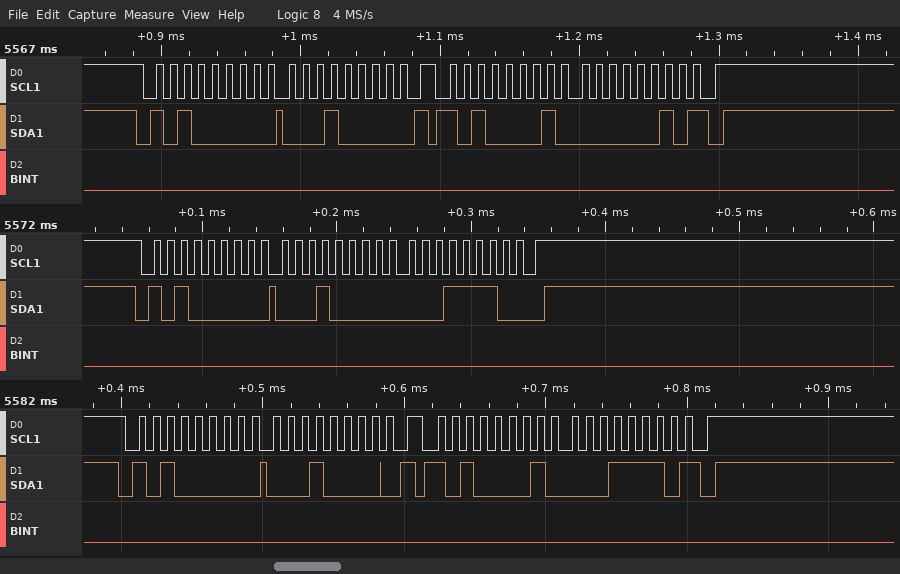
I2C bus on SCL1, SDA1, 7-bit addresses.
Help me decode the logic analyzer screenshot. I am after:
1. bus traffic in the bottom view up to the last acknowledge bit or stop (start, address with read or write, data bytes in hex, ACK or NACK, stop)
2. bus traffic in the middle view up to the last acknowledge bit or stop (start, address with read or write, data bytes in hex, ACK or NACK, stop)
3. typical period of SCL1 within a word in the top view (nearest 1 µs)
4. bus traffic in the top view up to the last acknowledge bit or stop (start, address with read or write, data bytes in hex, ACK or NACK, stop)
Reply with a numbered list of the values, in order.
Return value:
1. start, address 50 write ACK, 10 ACK, repeated start, address 50 read ACK, 1E NACK, stop
2. start, address 50 write ACK, 10 ACK, 1E ACK, stop
3. 10 µs
4. start, address 50 write ACK, 10 ACK, repeated start, address 50 read ACK, 02 NACK, stop
